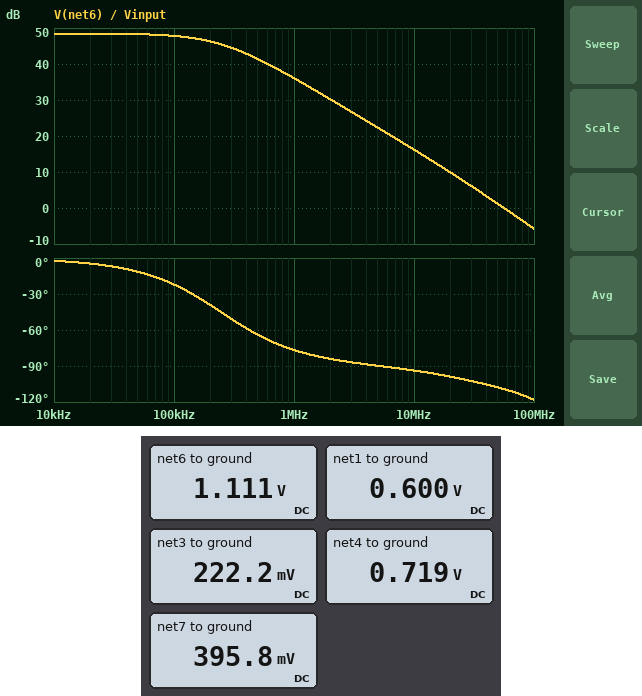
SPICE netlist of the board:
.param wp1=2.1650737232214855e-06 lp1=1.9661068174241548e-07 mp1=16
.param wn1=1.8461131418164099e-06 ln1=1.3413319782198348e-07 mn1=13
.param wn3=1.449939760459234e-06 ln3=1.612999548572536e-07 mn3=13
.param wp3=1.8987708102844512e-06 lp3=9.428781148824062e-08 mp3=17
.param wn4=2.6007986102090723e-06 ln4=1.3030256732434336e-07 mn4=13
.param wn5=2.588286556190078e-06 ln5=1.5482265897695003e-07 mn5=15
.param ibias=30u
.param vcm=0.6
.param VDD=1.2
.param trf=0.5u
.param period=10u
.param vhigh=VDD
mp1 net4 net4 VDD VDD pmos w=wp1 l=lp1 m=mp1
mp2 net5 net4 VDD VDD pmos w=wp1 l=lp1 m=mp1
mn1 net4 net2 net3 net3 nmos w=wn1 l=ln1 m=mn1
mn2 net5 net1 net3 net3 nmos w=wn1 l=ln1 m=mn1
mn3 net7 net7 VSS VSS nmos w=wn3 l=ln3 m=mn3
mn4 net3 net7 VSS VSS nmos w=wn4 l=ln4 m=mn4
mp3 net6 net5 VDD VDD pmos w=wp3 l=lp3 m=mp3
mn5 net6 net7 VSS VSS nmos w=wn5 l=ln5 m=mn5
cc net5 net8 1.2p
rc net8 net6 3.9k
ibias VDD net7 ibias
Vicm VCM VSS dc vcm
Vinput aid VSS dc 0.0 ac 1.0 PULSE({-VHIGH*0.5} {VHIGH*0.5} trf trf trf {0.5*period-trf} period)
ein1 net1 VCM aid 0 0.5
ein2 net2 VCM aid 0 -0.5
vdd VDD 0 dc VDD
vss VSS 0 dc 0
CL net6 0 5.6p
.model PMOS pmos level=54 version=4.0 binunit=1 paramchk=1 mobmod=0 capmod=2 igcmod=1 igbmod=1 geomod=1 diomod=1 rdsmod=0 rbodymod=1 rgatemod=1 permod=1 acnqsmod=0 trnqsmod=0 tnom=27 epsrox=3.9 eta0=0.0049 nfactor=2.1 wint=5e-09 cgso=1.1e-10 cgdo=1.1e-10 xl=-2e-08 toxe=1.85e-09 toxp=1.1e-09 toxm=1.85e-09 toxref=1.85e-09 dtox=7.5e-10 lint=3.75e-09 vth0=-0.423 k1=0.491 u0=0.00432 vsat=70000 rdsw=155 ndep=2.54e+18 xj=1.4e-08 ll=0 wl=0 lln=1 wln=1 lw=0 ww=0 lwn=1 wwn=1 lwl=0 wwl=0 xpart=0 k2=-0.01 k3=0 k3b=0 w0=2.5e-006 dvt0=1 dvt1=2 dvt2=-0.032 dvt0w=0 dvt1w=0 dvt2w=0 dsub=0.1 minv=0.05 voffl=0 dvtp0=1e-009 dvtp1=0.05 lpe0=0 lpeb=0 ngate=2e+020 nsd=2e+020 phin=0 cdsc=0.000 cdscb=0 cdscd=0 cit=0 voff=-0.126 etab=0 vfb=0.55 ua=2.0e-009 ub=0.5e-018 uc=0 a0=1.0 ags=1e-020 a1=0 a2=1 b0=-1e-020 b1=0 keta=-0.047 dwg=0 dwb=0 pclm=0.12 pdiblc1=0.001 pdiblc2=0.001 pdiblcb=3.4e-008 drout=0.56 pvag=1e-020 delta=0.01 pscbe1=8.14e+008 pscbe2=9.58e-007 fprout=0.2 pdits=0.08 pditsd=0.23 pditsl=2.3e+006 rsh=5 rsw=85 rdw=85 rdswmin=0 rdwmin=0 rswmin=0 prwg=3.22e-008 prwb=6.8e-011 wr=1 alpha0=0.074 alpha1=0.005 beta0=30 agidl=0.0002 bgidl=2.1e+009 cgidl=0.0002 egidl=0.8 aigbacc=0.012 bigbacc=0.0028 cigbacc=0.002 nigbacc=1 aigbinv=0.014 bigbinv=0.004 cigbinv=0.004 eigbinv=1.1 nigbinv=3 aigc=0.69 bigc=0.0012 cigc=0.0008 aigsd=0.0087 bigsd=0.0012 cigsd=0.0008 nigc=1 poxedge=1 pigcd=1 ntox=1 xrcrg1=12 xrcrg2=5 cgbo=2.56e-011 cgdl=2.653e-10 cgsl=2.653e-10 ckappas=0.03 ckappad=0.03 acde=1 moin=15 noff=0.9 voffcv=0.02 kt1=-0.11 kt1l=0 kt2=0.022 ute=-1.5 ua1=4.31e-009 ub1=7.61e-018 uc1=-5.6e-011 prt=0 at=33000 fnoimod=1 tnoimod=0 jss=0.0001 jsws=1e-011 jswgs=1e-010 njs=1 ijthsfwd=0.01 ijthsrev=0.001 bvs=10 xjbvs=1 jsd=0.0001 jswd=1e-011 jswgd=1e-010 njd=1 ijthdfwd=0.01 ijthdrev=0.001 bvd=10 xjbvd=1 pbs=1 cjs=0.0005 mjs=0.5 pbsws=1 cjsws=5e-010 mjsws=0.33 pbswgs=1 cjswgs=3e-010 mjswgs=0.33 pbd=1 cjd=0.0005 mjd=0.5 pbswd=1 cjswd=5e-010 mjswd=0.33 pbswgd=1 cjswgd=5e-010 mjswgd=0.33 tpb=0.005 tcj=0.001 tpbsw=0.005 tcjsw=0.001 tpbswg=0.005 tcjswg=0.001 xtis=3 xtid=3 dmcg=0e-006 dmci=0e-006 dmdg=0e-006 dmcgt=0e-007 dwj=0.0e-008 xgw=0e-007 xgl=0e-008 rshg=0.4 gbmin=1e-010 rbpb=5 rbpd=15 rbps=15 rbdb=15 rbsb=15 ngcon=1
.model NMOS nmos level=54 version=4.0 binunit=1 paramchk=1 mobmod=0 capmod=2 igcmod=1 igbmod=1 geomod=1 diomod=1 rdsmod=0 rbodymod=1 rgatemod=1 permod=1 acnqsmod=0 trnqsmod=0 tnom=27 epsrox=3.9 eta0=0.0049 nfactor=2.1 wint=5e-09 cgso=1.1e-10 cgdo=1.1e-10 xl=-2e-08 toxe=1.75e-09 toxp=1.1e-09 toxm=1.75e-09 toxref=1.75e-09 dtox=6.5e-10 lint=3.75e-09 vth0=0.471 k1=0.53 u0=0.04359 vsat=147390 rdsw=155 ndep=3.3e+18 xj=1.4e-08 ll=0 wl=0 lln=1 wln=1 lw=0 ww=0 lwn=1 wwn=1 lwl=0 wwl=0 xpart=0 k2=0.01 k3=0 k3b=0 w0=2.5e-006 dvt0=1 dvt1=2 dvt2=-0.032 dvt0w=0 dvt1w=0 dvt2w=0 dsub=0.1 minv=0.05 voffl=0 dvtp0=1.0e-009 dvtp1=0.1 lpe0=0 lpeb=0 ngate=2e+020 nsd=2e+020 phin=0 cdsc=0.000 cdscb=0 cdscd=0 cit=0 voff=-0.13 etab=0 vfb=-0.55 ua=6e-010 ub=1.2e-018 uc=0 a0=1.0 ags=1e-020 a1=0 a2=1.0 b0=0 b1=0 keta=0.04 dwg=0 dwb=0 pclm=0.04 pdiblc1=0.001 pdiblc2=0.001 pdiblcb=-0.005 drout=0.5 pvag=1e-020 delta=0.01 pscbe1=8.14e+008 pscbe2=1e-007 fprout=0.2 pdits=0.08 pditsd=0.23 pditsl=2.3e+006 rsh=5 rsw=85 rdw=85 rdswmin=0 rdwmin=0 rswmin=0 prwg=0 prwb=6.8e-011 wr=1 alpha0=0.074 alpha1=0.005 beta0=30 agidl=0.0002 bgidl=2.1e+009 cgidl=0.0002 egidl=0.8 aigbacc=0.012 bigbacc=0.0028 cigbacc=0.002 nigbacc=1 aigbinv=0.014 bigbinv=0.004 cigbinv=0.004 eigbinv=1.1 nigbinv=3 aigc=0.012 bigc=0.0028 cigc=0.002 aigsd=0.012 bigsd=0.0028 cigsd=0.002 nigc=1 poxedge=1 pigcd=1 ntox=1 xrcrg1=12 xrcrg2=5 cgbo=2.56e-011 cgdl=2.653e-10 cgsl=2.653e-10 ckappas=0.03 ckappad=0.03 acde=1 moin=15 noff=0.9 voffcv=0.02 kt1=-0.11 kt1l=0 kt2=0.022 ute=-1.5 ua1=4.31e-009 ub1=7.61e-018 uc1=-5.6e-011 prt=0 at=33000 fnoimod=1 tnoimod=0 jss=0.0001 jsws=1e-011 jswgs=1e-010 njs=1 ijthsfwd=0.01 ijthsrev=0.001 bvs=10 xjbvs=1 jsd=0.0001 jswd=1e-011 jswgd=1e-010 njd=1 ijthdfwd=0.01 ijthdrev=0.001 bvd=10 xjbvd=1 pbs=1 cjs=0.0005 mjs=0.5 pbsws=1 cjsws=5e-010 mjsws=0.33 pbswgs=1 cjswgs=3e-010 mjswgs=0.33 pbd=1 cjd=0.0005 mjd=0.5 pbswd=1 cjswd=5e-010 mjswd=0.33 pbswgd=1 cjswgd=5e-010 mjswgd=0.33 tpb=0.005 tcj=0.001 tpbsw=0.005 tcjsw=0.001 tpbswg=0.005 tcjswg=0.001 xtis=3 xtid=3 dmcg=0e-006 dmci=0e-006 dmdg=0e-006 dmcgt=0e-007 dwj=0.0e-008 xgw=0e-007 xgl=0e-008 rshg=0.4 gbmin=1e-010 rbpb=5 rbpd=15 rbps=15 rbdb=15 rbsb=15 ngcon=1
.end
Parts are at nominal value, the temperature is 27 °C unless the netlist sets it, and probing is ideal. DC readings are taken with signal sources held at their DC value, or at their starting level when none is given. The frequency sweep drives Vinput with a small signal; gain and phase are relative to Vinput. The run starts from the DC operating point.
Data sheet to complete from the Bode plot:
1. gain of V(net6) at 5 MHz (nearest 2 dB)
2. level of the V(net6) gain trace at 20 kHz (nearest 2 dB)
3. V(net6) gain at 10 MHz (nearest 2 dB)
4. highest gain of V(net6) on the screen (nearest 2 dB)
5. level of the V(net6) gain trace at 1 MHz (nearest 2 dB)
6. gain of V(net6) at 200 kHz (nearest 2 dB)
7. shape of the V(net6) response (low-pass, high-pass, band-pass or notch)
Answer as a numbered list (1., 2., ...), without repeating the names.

1. 22 dB
2. 48 dB
3. 16 dB
4. 48 dB
5. 36 dB
6. 46 dB
7. low-pass
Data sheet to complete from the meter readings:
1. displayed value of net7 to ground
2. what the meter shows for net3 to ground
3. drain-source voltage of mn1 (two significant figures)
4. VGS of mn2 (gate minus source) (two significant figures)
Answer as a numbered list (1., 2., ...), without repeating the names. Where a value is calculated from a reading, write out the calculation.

1. 395.8 mV
2. 222.2 mV
3. 719 mV - 222.2 mV = 500 mV
4. 600 mV - 222.2 mV = 380 mV
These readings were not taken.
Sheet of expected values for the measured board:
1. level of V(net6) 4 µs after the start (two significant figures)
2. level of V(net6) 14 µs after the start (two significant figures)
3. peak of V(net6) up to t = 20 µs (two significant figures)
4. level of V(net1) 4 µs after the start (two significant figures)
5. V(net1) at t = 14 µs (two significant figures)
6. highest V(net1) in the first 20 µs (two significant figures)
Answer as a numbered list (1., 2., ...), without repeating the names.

1. 1.2 V
2. 1.2 V
3. 1.2 V
4. 900 mV
5. 900 mV
6. 900 mV
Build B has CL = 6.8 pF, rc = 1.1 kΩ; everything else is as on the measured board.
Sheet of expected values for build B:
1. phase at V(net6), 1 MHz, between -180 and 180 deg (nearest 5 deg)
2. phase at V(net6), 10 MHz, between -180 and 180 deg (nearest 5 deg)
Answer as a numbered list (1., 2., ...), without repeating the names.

1. -80 deg
2. -110 deg
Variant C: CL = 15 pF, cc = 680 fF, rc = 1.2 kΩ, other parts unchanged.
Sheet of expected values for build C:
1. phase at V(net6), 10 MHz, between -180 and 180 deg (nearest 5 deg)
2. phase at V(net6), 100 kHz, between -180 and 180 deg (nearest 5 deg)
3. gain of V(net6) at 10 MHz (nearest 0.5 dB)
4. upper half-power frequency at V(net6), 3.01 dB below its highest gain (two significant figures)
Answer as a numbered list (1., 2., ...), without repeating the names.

1. -125 deg
2. -15 deg
3. 18.5 dB
4. 400 kHz
